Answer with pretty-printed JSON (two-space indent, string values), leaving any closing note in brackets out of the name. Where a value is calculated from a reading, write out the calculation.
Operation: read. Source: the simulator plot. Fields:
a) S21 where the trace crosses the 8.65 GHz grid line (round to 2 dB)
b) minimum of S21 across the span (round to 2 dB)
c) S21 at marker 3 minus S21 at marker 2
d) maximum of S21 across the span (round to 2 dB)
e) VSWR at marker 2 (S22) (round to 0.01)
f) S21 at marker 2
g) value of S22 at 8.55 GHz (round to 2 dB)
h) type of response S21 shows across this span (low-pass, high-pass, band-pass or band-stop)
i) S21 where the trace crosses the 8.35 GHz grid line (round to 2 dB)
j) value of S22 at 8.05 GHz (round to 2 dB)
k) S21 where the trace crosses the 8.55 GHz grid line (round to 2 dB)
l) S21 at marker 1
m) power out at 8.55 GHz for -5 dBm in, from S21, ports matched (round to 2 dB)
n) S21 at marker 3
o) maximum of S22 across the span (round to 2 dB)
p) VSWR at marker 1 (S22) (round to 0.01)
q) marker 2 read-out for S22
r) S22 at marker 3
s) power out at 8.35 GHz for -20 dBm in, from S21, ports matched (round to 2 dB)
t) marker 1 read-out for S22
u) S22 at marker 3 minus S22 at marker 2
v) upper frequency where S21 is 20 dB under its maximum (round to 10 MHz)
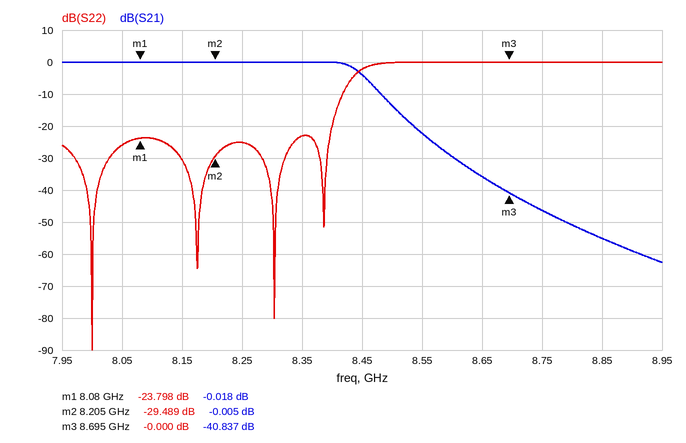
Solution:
{
  "S21 where the trace crosses the 8.65 GHz grid line": "-36 dB",
  "minimum of S21 across the span": "-62 dB",
  "S21 at marker 3 minus S21 at marker 2": "-40.837 − (-0.005) = -40.832 dB",
  "maximum of S21 across the span": "0 dB",
  "VSWR at marker 2 (S22)": "(1 + 0.0335)/(1 − 0.0335) ≈ 1.07",
  "S21 at marker 2": "-0.005 dB",
  "value of S22 at 8.55 GHz": "0 dB",
  "type of response S21 shows across this span": "low-pass",
  "S21 where the trace crosses the 8.35 GHz grid line": "0 dB",
  "value of S22 at 8.05 GHz": "-26 dB",
  "S21 where the trace crosses the 8.55 GHz grid line": "-22 dB",
  "S21 at marker 1": "-0.018 dB",
  "power out at 8.55 GHz for -5 dBm in, from S21, ports matched": "-5 dBm + (-22 dB) = -28 dBm",
  "S21 at marker 3": "-40.837 dB",
  "maximum of S22 across the span": "0 dB",
  "VSWR at marker 1 (S22)": "(1 + 0.0646)/(1 − 0.0646) ≈ 1.14",
  "marker 2 read-out for S22": "-29.489 dB",
  "S22 at marker 3": "-0.000 dB",
  "power out at 8.35 GHz for -20 dBm in, from S21, ports matched": "-20 dBm + (0 dB) = -20 dBm",
  "marker 1 read-out for S22": "-23.798 dB",
  "S22 at marker 3 minus S22 at marker 2": "-0 − (-29.489) = 29.489 dB",
  "upper frequency where S21 is 20 dB under its maximum": "8.54 GHz"
}
